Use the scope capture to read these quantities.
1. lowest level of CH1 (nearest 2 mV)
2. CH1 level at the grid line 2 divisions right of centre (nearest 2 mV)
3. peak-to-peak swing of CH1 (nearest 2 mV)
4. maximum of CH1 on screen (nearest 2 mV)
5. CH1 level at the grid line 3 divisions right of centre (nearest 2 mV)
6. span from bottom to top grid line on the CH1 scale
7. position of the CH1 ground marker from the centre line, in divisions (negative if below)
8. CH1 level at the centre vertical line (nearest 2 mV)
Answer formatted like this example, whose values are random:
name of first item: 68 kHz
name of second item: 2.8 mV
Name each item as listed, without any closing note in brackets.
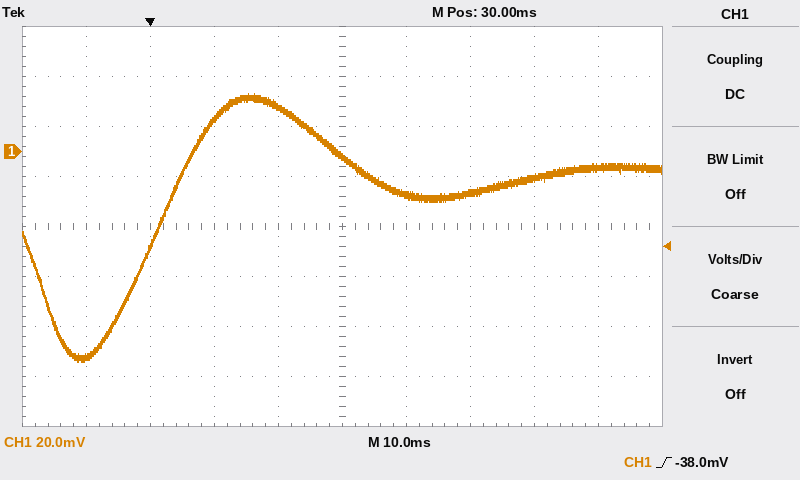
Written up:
lowest level of CH1: -84 mV
CH1 level at the grid line 2 divisions right of centre: -16 mV
peak-to-peak swing of CH1: 108 mV
maximum of CH1 on screen: 24 mV
CH1 level at the grid line 3 divisions right of centre: -10 mV
span from bottom to top grid line on the CH1 scale: 160 mV
position of the CH1 ground marker from the centre line, in divisions: +1.5 div
CH1 level at the centre vertical line: -2 mV
